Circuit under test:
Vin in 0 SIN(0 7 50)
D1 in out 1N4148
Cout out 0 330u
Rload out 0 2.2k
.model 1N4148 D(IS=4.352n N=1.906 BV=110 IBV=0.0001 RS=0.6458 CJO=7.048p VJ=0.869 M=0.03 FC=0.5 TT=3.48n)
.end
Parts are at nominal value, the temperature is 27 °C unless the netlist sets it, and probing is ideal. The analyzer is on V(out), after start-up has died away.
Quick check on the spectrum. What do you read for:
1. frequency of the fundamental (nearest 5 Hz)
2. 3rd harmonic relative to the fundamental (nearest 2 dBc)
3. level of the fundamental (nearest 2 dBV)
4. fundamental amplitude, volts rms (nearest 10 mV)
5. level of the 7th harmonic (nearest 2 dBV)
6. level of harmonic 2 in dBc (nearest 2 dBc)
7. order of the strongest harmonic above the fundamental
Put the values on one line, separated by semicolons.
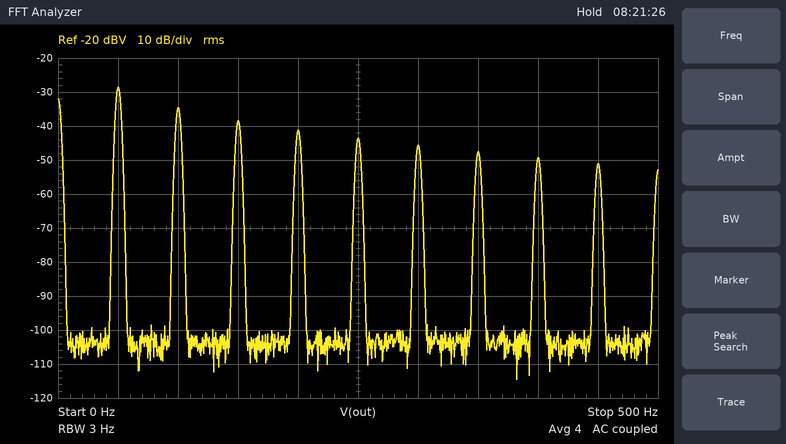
50 Hz; -10 dBc; -28 dBV; 40 mV; -48 dBV; -6 dBc; 2
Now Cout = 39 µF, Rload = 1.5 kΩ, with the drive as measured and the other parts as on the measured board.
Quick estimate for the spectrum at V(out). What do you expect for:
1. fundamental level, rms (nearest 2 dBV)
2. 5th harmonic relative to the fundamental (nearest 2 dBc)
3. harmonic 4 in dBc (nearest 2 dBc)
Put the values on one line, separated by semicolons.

-8 dBV; -18 dBc; -14 dBc
